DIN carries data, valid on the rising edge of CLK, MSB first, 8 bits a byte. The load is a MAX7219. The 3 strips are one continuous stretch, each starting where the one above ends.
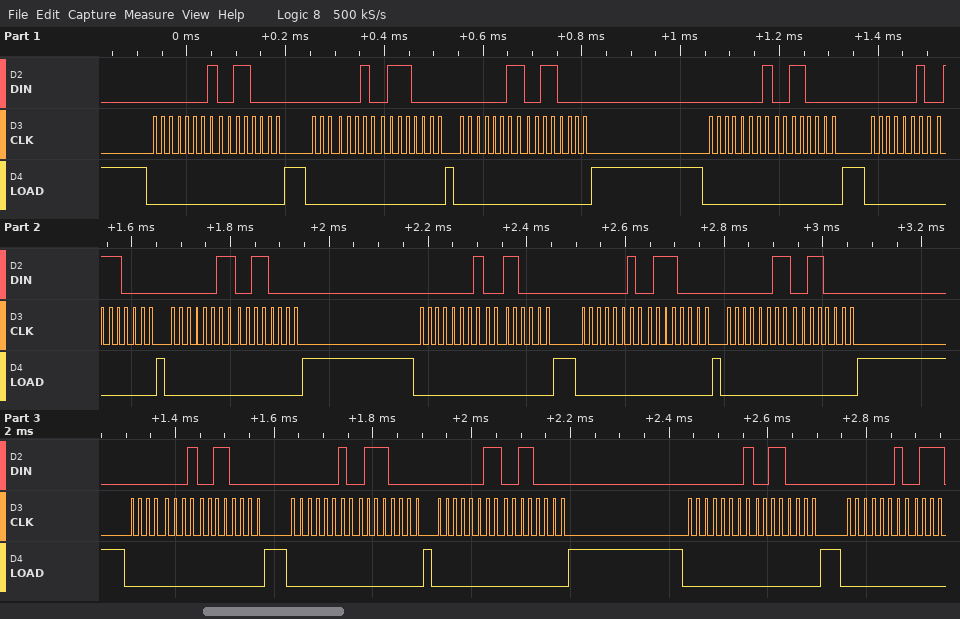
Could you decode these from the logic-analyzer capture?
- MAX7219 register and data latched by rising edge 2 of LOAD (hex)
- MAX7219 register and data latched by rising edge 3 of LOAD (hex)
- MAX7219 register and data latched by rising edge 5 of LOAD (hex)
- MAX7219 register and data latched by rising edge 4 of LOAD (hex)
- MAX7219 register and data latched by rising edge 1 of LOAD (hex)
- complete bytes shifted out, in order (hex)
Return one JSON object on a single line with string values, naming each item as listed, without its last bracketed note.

{"MAX7219 register and data latched by rising edge 2 of LOAD": "register 0x2, data 0x70", "MAX7219 register and data latched by rising edge 3 of LOAD": "register 0x3, data 0x30", "MAX7219 register and data latched by rising edge 5 of LOAD": "register 0x2, data 0x70", "MAX7219 register and data latched by rising edge 4 of LOAD": "register 0x1, data 0x30", "MAX7219 register and data latched by rising edge 1 of LOAD": "register 0x1, data 0x30", "complete bytes shifted out, in order": "01 30 02 70 03 30 01 30 02 70 03 30 01 30 02 70 03 30 01 30 02 70 03 30 01 30 02"}
